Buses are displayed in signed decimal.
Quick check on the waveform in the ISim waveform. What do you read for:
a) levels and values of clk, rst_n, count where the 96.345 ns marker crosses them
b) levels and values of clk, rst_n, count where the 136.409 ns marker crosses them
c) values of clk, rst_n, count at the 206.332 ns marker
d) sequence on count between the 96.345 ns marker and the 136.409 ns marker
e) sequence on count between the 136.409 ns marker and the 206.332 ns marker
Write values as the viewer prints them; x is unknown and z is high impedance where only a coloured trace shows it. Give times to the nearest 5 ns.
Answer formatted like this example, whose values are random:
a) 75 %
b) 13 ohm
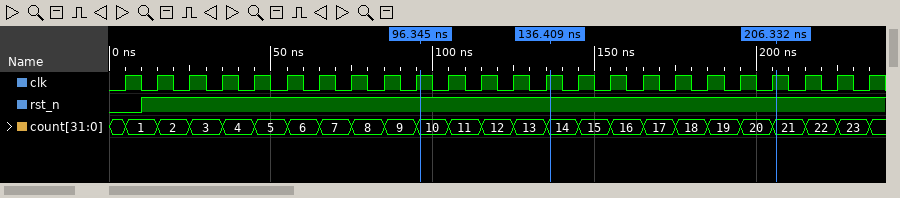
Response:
a) clk=1, rst_n=1, count=10
b) clk=1, rst_n=1, count=14
c) clk=1, rst_n=1, count=21
d) 10, 11, 12, 13, 14
e) 14, 15, 16, 17, 18, 19, 20, 21
